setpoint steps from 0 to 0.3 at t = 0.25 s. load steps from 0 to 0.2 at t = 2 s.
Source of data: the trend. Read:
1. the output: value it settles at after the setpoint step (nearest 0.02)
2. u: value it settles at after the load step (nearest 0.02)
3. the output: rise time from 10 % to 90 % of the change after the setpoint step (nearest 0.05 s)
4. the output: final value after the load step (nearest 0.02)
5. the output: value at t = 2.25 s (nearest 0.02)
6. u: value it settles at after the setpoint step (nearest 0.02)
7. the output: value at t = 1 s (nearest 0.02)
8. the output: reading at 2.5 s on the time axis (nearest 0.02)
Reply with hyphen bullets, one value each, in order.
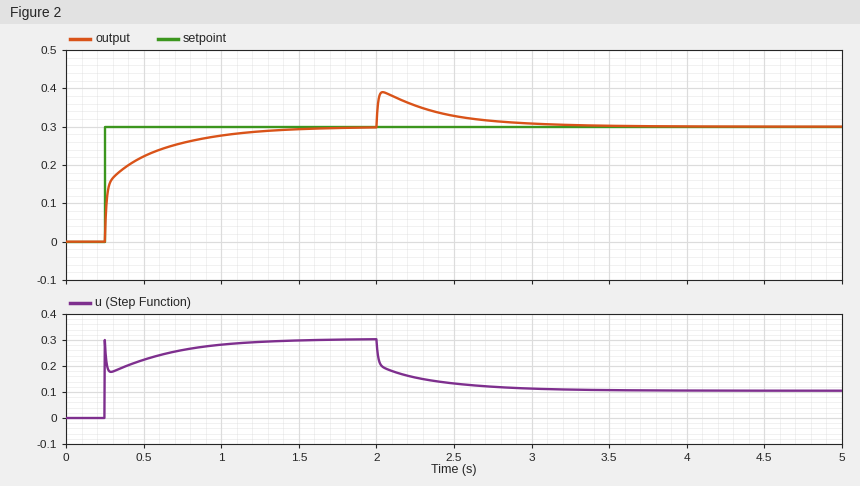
- 0.30
- 0.10
- 0.65 s
- 0.30
- 0.36
- 0.30
- 0.28
- 0.32
